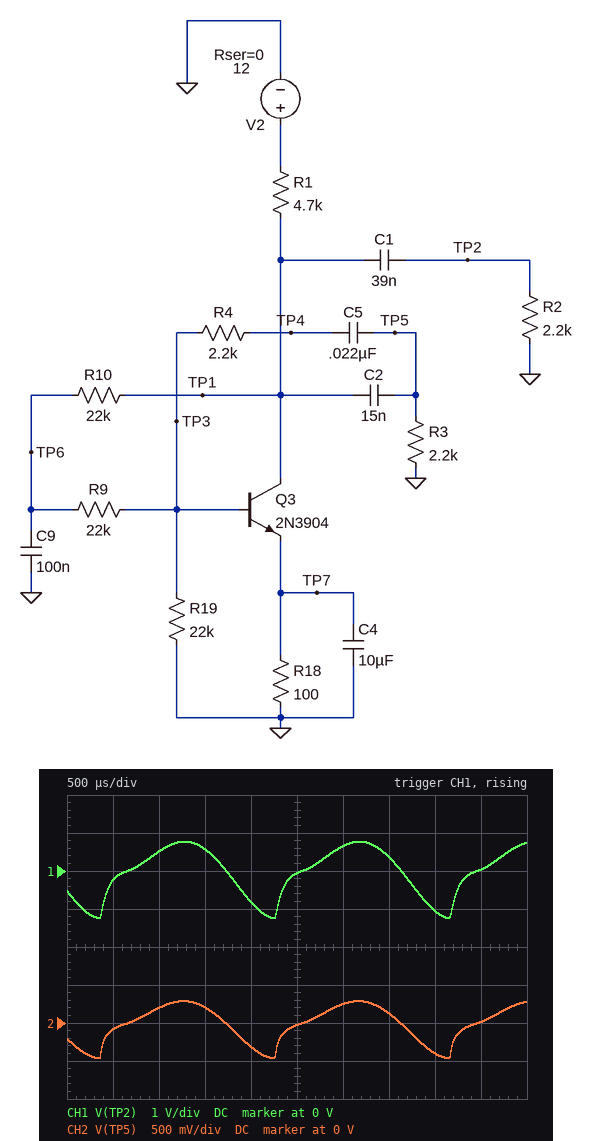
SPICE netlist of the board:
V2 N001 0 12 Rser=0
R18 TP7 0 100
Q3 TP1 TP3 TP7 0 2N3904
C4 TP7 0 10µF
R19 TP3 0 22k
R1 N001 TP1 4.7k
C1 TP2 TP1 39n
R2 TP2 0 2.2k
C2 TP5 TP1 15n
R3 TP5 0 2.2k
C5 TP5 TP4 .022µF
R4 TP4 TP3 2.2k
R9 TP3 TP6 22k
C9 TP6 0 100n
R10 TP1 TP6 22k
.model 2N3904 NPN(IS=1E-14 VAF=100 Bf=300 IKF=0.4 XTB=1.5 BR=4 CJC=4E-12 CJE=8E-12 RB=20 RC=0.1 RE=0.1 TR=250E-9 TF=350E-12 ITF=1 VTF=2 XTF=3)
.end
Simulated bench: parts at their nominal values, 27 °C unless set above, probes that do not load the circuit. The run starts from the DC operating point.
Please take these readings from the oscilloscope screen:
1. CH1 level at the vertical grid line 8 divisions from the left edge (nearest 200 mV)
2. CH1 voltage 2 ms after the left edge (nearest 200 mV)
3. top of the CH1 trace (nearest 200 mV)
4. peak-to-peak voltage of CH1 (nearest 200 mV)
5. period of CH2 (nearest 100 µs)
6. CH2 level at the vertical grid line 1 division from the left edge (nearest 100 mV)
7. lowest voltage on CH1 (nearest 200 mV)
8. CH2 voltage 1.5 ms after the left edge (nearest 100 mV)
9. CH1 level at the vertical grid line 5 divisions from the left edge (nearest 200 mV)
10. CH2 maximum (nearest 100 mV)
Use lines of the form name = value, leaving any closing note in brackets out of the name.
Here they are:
CH1 level at the vertical grid line 8 divisions from the left edge = -1.0 V
CH1 voltage 2 ms after the left edge = -800 mV
top of the CH1 trace = 800 mV
peak-to-peak voltage of CH1 = 2.0 V
period of CH2 = 1.9 ms
CH2 level at the vertical grid line 1 division from the left edge = -100 mV
lowest voltage on CH1 = -1.2 V
CH2 voltage 1.5 ms after the left edge = 200 mV
CH1 level at the vertical grid line 5 divisions from the left edge = 0 V
CH2 maximum = 300 mV
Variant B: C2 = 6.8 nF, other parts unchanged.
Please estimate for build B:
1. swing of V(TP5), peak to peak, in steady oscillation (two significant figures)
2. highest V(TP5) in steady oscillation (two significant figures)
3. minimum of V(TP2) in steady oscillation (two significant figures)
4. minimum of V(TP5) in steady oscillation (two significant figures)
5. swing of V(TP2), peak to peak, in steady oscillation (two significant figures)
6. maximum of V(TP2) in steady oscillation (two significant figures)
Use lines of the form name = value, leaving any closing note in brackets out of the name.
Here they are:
swing of V(TP5), peak to peak, in steady oscillation = 380 mV
highest V(TP5) in steady oscillation = 160 mV
minimum of V(TP2) in steady oscillation = -1.3 V
minimum of V(TP5) in steady oscillation = -220 mV
swing of V(TP2), peak to peak, in steady oscillation = 2.3 V
maximum of V(TP2) in steady oscillation = 950 mV
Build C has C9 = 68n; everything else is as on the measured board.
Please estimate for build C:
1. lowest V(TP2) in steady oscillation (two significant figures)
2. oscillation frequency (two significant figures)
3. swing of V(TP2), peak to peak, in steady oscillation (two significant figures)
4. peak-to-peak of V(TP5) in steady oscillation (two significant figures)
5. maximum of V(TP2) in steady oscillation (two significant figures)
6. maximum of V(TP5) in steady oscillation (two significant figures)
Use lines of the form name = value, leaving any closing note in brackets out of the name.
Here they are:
lowest V(TP2) in steady oscillation = -1.4 V
oscillation frequency = 590 Hz
swing of V(TP2), peak to peak, in steady oscillation = 2.2 V
peak-to-peak of V(TP5) in steady oscillation = 830 mV
maximum of V(TP2) in steady oscillation = 870 mV
maximum of V(TP5) in steady oscillation = 320 mV
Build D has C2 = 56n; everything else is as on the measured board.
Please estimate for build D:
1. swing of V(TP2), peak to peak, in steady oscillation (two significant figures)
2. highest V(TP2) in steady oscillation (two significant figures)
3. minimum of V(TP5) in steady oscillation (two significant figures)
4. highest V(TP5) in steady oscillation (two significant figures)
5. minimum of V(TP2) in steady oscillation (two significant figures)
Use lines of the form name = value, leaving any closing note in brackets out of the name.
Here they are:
swing of V(TP2), peak to peak, in steady oscillation = 1.3 V
highest V(TP2) in steady oscillation = 500 mV
minimum of V(TP5) in steady oscillation = -1.1 V
highest V(TP5) in steady oscillation = 690 mV
minimum of V(TP2) in steady oscillation = -790 mV
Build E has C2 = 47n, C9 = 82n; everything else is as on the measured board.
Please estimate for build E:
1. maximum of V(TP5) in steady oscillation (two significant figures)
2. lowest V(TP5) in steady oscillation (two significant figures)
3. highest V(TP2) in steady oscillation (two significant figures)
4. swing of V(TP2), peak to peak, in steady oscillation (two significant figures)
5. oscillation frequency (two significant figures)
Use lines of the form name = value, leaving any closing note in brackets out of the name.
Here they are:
maximum of V(TP5) in steady oscillation = 650 mV
lowest V(TP5) in steady oscillation = -1.0 V
highest V(TP2) in steady oscillation = 570 mV
swing of V(TP2), peak to peak, in steady oscillation = 1.4 V
oscillation frequency = 380 Hz
